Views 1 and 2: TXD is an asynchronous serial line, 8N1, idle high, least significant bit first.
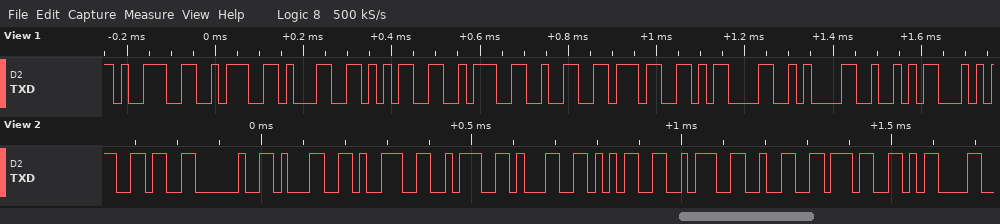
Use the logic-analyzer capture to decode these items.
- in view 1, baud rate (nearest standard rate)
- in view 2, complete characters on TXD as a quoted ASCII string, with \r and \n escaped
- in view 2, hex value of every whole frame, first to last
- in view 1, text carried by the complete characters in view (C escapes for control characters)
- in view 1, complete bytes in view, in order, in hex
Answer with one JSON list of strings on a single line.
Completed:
["57600 baud", "\"6 19:15:27\\r\"", "36 20 31 39 3A 31 35 3A 32 37 0D", "\"9:15:27\\r\\nR\"", "39 3A 31 35 3A 32 37 0D 0A 52"]
